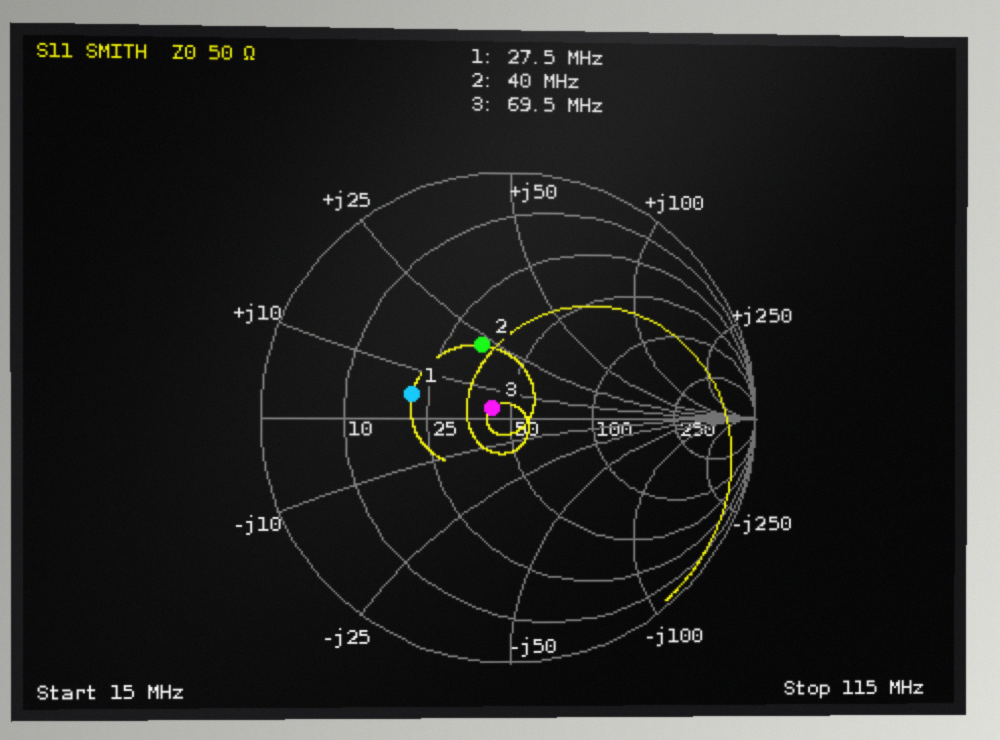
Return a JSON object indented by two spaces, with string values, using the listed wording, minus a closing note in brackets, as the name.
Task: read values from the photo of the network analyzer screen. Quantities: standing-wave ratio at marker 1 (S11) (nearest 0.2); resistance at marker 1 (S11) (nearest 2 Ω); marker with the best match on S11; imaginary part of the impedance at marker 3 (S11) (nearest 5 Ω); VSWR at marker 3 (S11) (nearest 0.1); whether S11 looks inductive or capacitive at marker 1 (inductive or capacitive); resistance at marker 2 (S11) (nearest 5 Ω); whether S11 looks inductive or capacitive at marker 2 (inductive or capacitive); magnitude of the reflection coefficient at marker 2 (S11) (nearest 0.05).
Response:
{
  "standing-wave ratio at marker 1 (S11)": "2.4",
  "resistance at marker 1 (S11)": "22 Ω",
  "marker with the best match on S11": "marker 3",
  "imaginary part of the impedance at marker 3 (S11)": "+5 Ω",
  "VSWR at marker 3 (S11)": "1.2",
  "whether S11 looks inductive or capacitive at marker 1": "inductive",
  "resistance at marker 2 (S11)": "35 Ω",
  "whether S11 looks inductive or capacitive at marker 2": "inductive",
  "magnitude of the reflection coefficient at marker 2 (S11)": "0.30"
}
